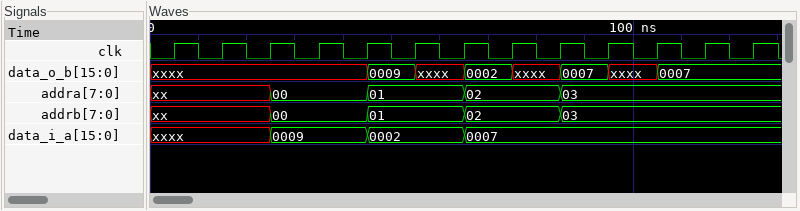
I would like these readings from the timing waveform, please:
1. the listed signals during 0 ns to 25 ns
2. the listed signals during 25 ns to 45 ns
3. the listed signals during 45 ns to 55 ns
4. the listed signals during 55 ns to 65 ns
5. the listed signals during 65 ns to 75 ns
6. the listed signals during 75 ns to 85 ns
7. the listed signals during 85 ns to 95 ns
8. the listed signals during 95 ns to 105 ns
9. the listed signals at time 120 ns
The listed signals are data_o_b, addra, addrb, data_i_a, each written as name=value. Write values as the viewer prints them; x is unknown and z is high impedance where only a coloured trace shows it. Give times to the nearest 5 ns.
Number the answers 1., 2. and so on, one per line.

1. data_o_b=xxxx, addra=xx, addrb=xx, data_i_a=xxxx
2. data_o_b=xxxx, addra=00, addrb=00, data_i_a=0009
3. data_o_b=0009, addra=01, addrb=01, data_i_a=0002
4. data_o_b=xxxx, addra=01, addrb=01, data_i_a=0002
5. data_o_b=0002, addra=02, addrb=02, data_i_a=0007
6. data_o_b=xxxx, addra=02, addrb=02, data_i_a=0007
7. data_o_b=0007, addra=03, addrb=03, data_i_a=0007
8. data_o_b=xxxx, addra=03, addrb=03, data_i_a=0007
9. data_o_b=0007, addra=03, addrb=03, data_i_a=0007
